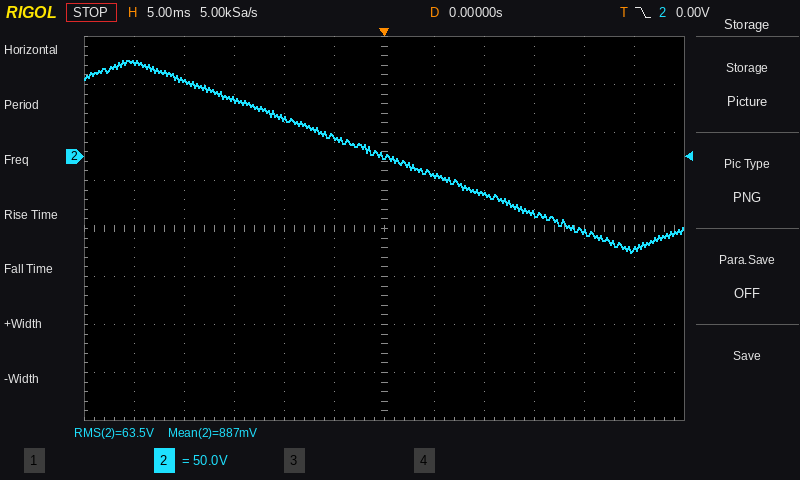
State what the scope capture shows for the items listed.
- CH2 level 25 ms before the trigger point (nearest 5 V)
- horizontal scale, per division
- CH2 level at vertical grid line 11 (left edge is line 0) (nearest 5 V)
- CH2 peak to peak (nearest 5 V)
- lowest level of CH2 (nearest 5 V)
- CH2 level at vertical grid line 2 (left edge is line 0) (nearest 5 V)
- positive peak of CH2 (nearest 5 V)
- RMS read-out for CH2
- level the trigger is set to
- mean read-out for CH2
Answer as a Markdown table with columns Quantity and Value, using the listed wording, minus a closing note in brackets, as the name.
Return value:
| Quantity | Value |
|---|---|
| CH2 level 25 ms before the trigger point | 100 V |
| horizontal scale, per division | 5 ms |
| CH2 level at vertical grid line 11 (left edge is line 0) | -95 V |
| CH2 peak to peak | 200 V |
| lowest level of CH2 | -100 V |
| CH2 level at vertical grid line 2 (left edge is line 0) | 80 V |
| positive peak of CH2 | 100 V |
| RMS read-out for CH2 | 63.5 V |
| level the trigger is set to | 0.00 V |
| mean read-out for CH2 | 887 mV |
